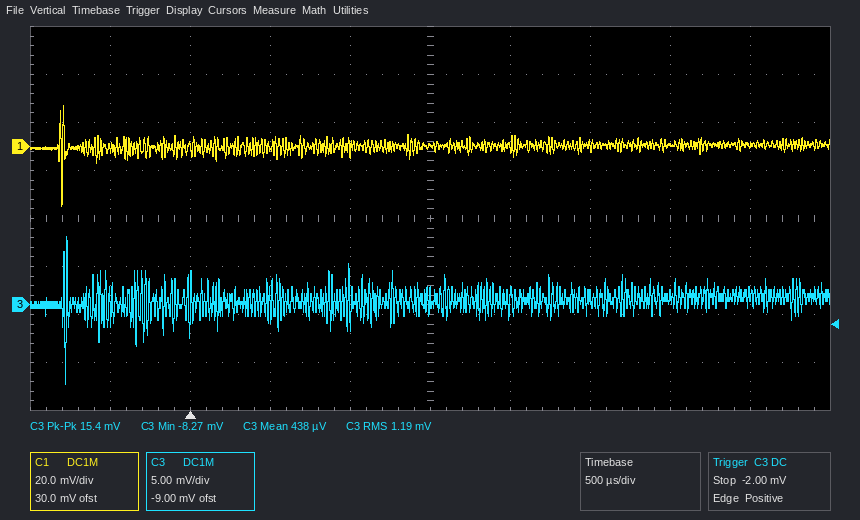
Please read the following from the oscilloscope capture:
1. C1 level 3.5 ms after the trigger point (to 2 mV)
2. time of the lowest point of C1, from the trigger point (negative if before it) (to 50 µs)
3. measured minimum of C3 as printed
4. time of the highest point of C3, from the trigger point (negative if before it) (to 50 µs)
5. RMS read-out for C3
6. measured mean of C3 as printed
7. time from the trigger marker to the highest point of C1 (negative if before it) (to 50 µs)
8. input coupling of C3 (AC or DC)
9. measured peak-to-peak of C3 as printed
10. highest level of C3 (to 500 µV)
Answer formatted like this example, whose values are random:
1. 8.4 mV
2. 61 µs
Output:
1. 0 mV
2. -800 µs
3. -8.27 mV
4. -750 µs
5. 1.19 mV
6. 438 µV
7. -800 µs
8. DC
9. 15.4 mV
10. 7.0 mV
